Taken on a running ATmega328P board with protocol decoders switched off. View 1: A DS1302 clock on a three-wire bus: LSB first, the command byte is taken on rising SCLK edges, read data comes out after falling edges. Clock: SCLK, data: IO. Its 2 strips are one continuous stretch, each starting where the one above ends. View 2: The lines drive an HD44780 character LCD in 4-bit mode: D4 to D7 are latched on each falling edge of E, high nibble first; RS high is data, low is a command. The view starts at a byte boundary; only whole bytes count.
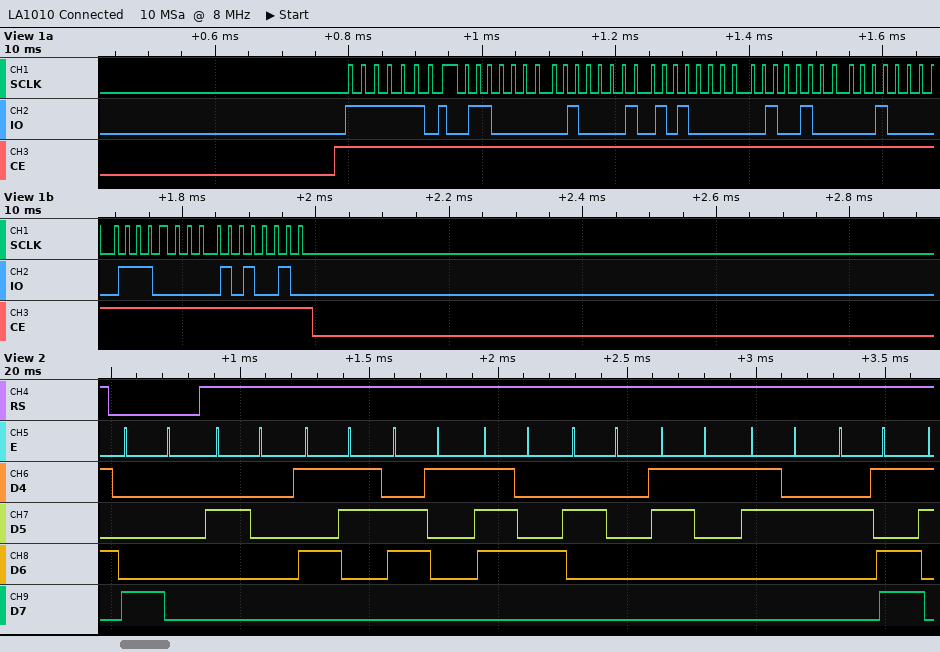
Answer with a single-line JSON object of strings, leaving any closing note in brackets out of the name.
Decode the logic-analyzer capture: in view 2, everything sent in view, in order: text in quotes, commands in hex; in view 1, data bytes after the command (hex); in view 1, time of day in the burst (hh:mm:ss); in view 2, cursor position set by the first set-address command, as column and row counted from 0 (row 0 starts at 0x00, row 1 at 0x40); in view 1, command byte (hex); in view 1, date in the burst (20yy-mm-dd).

{"in view 2, everything sent in view, in order: text in quotes, commands in hex": "0x80 \" Sat 12-\"", "in view 1, data bytes after the command": "06 42 05 12 04 07 25", "in view 1, time of day in the burst": "05:42:06", "in view 2, cursor position set by the first set-address command, as column and row counted from 0": "column 0, row 0", "in view 1, command byte": "0xBF", "in view 1, date in the burst": "2025-04-12"}
